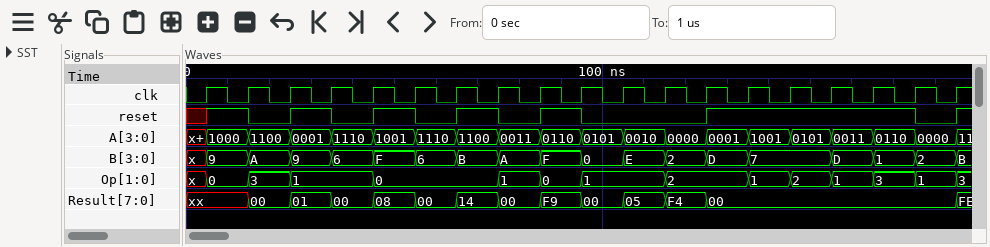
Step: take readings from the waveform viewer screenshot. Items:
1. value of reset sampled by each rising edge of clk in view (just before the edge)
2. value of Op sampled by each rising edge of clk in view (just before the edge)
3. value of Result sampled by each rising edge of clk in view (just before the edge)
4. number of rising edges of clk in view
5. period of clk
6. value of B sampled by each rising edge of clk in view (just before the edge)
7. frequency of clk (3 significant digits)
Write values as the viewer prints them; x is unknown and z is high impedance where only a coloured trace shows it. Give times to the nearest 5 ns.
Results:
x 1 0 1 0 1 0 1 0 1 0 0 0 1 1 1 1 1 0
x, 0, 3, 1, 1, 0, 0, 0, 1, 0, 1, 1, 2, 2, 1, 2, 1, 3, 1
xx, xx, 00, 01, 00, 08, 00, 14, 00, F9, 00, 05, F4, 00, 00, 00, 00, 00, 00
19
10 ns
x, 9, A, 9, 6, F, 6, B, A, F, 0, E, 2, D, 7, 7, D, 1, 2
100 MHz
